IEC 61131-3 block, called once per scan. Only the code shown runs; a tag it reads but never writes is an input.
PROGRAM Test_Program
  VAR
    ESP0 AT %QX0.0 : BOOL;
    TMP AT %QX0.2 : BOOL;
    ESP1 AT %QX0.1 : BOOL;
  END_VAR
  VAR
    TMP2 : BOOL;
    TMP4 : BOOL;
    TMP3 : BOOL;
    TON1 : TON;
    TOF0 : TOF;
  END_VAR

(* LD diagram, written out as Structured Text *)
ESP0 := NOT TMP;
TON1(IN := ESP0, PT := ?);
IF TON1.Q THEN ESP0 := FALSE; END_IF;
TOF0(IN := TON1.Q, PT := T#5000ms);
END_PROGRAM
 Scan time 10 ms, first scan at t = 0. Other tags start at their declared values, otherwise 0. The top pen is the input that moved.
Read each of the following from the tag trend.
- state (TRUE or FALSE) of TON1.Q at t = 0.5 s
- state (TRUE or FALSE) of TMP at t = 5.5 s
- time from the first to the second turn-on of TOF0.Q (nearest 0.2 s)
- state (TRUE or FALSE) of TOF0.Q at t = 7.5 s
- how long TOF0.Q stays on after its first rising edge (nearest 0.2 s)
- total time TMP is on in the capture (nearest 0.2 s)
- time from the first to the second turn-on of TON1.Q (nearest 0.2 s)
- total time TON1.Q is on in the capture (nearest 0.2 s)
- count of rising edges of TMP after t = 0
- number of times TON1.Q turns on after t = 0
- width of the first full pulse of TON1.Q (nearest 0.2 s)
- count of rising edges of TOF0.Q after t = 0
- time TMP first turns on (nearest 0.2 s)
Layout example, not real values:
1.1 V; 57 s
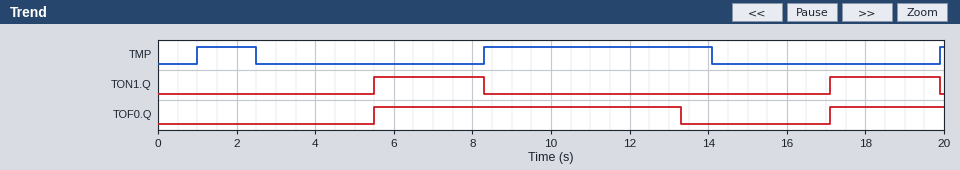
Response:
FALSE; FALSE; 11.6 s; TRUE; 7.8 s; 7.4 s; 11.6 s; 5.6 s; 3; 2; 2.8 s; 2; 1.0 s
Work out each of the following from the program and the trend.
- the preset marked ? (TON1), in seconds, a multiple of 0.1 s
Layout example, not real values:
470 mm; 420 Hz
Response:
3.0 s
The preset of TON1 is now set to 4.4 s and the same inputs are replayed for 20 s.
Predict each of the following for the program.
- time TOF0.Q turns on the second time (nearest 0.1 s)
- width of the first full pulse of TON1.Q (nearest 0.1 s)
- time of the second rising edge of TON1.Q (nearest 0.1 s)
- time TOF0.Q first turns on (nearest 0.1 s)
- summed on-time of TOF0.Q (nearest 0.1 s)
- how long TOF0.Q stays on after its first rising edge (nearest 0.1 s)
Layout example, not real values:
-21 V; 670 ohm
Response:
18.5 s; 1.4 s; 18.5 s; 6.9 s; 7.9 s; 6.4 s
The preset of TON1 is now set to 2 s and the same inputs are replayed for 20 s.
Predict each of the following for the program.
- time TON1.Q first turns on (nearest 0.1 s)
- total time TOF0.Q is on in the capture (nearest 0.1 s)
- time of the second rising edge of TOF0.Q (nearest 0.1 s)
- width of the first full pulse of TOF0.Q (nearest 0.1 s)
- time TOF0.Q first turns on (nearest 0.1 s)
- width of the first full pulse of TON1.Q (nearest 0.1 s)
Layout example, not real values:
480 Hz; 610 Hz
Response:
4.5 s; 12.7 s; 16.1 s; 8.8 s; 4.5 s; 3.8 s
